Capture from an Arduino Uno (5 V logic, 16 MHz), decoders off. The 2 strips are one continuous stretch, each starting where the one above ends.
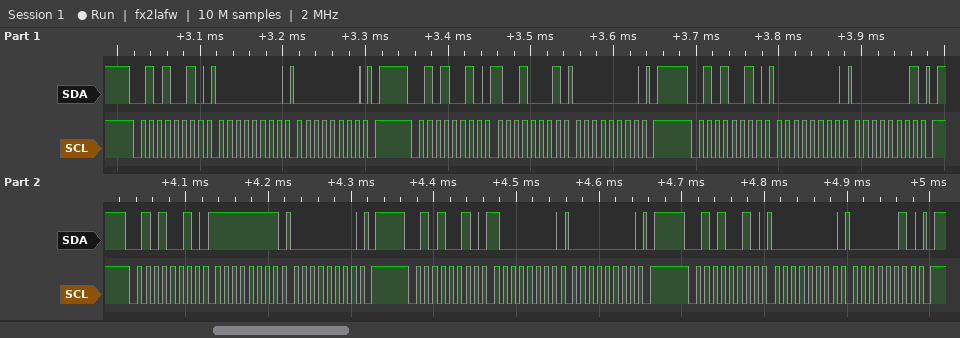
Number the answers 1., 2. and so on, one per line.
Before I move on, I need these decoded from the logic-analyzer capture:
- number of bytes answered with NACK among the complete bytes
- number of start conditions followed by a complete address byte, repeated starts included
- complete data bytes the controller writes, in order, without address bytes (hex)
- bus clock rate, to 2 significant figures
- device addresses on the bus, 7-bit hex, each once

1. 0
2. 6
3. 00 00 91 00 00 01 FF 00 80 00 00 02
4. 100 kHz
5. 0x29
